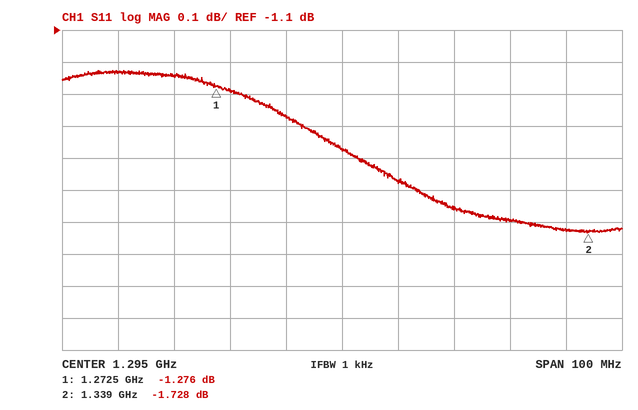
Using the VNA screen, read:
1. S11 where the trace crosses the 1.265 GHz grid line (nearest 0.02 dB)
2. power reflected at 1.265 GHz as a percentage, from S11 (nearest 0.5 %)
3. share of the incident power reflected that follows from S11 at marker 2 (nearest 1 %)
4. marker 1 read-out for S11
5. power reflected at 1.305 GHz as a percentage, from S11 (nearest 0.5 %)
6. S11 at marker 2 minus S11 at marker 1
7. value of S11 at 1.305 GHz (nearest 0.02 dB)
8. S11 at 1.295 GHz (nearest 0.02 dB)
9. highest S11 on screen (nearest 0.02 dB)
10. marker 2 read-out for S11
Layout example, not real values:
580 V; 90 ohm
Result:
-1.24 dB; 75.0 %; 67 %; -1.276 dB; 69.5 %; -0.452 dB; -1.58 dB; -1.48 dB; -1.22 dB; -1.728 dB
